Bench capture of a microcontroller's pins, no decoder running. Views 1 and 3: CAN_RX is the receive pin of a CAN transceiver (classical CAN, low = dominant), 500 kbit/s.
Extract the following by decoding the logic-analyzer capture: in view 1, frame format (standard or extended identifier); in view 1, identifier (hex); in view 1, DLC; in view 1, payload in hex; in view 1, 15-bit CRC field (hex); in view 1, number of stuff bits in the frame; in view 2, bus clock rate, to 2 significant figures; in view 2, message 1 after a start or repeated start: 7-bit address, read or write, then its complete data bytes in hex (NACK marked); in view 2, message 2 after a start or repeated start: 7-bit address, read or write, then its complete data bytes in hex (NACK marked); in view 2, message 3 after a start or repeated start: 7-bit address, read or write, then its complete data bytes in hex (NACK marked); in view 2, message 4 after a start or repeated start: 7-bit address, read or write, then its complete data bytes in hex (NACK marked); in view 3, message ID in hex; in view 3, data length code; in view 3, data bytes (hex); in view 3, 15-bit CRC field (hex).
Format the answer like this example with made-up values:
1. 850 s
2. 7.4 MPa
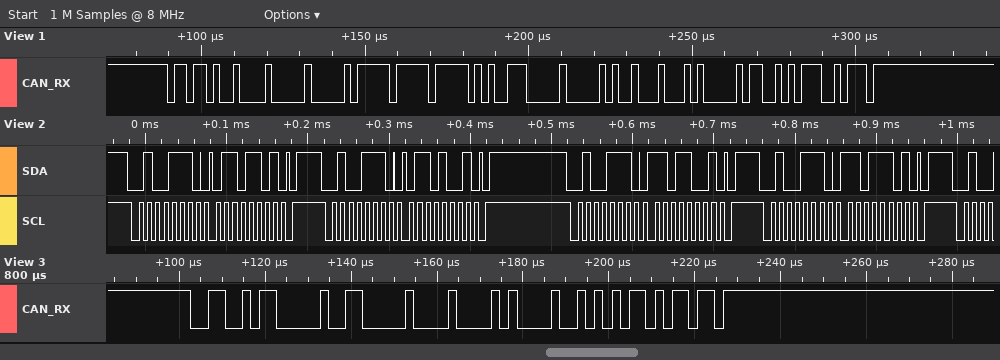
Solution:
1. standard
2. 0x6D2
3. 8
4. 00 FF FF 4E 00 24 45 03
5. 0x15CB
6. 8
7. 100 kHz
8. 0x27 write: 6D
9. 0x27 write: 69
10. 0x27 write: D9
11. 0x27 write: DD
12. 0x32C
13. 3
14. 00 42 84
15. 0x55AD
